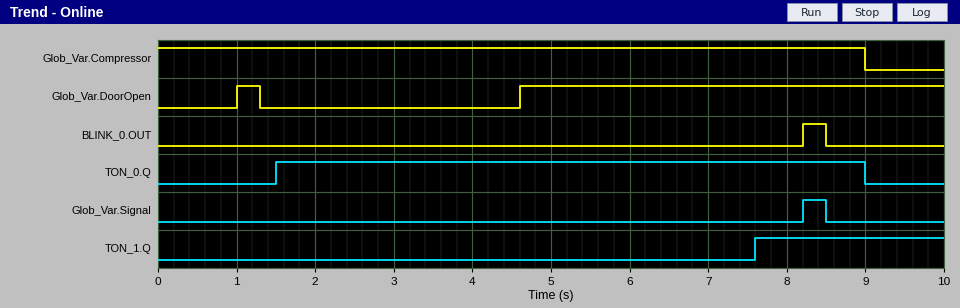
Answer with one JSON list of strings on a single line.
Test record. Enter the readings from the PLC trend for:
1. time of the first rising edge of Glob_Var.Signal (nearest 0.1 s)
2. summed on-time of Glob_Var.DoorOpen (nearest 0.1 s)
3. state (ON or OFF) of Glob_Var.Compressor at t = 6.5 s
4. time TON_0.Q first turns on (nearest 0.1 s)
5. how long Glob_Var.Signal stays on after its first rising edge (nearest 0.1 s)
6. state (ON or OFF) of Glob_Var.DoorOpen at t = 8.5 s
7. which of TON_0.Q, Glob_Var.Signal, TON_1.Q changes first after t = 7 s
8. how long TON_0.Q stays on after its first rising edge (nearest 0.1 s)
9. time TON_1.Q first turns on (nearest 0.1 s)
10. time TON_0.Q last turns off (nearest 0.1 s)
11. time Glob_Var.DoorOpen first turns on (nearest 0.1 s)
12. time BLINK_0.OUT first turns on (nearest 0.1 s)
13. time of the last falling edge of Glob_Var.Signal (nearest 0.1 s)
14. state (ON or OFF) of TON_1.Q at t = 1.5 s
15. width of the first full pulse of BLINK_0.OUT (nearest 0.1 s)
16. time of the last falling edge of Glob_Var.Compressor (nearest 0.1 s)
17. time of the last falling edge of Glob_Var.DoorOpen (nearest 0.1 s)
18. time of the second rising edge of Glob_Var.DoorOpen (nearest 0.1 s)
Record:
["8.2 s", "5.7 s", "ON", "1.5 s", "0.3 s", "ON", "TON_1.Q", "7.5 s", "7.6 s", "9.0 s", "1.0 s", "8.2 s", "8.5 s", "OFF", "0.3 s", "9.0 s", "1.3 s", "4.6 s"]
